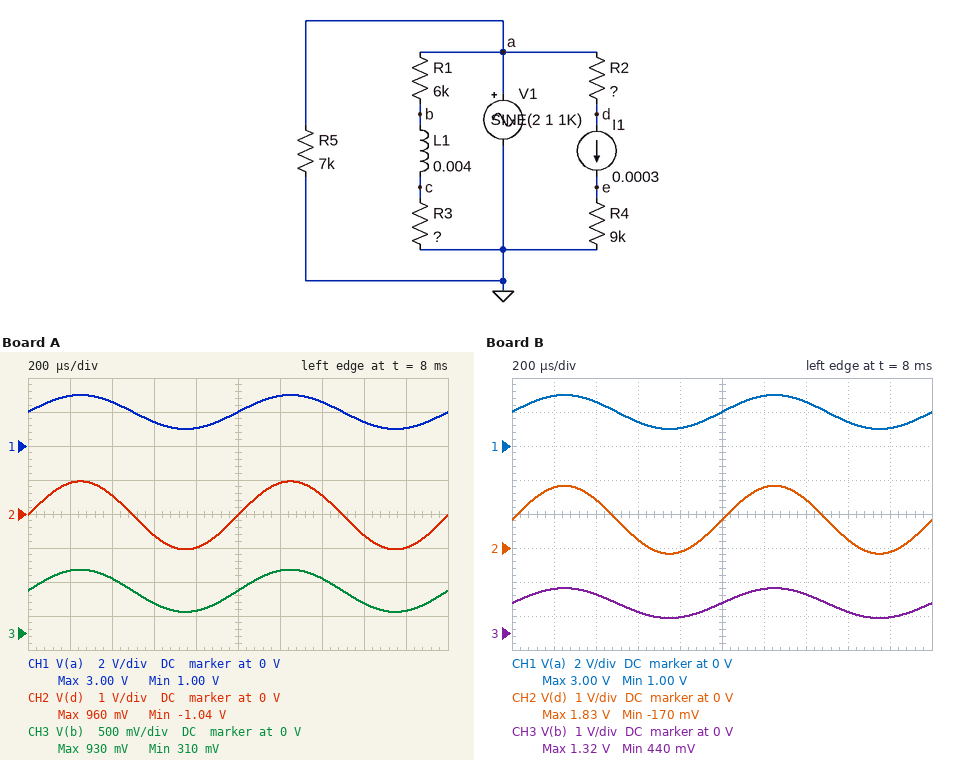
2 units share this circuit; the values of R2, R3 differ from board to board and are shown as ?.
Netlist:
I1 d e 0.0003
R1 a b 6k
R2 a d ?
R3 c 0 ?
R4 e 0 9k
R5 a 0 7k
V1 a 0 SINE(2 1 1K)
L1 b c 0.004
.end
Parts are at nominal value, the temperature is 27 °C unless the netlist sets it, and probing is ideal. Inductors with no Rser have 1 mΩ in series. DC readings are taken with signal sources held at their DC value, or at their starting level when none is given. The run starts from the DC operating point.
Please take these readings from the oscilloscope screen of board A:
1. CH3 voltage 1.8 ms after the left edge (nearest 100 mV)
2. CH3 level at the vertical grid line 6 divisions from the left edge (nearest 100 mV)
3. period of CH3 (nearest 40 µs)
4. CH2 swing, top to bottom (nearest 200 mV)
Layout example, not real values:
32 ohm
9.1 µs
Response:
300 mV
900 mV
1.00 ms
2.0 V
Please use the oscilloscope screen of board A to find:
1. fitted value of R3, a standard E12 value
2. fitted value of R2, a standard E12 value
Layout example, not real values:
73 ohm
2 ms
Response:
2.7 kΩ
6.8 kΩ
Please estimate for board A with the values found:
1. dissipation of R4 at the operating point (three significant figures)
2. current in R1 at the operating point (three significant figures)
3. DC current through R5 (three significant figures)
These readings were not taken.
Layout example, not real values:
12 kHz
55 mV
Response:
810 µW
230 µA
286 µA
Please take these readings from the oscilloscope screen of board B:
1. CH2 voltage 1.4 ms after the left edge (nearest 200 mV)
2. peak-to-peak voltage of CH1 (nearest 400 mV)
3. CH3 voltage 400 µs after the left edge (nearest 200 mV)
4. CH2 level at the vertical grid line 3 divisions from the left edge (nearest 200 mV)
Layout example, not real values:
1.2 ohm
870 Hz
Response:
1.4 V
2.0 V
1.2 V
200 mV
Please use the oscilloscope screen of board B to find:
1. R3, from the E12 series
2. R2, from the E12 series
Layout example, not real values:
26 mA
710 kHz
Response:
4.7 kΩ
3.9 kΩ
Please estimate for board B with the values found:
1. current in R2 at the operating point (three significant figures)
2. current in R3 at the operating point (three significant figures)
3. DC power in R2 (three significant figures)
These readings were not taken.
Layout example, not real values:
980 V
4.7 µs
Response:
300 µA
187 µA
351 µW
